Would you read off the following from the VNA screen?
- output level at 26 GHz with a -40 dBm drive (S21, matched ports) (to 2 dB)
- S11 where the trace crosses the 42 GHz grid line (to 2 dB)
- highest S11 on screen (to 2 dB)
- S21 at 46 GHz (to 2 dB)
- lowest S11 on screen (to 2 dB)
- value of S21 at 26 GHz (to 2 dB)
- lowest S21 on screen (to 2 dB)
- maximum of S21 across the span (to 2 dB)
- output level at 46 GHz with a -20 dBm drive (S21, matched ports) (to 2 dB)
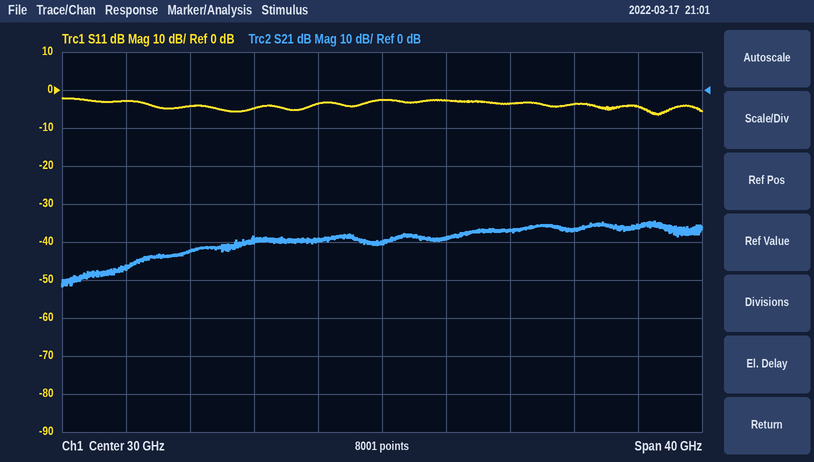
-80 dBm
-4 dB
-2 dB
-36 dB
-6 dB
-40 dB
-52 dB
-34 dB
-56 dBm
